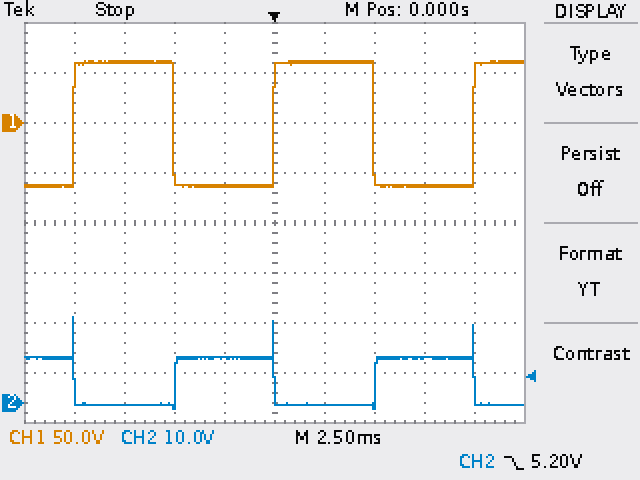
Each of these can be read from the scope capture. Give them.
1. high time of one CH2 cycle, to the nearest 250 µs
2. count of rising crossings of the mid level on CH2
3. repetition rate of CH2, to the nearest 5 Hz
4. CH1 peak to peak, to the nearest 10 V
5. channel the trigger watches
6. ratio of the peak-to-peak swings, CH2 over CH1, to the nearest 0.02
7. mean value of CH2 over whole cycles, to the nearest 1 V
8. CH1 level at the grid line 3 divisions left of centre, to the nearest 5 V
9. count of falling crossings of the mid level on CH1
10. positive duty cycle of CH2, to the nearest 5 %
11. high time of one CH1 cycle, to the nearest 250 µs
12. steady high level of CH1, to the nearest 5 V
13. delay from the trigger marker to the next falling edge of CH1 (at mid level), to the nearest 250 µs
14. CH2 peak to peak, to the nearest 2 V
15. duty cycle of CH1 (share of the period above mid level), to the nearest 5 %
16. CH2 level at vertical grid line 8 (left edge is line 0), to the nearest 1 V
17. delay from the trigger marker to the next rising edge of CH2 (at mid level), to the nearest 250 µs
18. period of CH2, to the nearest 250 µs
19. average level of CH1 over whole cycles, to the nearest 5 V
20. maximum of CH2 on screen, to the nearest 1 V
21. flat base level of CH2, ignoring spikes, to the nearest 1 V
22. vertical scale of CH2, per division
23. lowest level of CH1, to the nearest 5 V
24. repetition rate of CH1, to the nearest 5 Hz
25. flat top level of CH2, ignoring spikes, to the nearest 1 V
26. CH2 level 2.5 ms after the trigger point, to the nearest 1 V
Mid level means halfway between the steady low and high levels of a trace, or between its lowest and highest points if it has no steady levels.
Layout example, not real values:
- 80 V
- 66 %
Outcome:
- 5.00 ms
- 2
- 100 Hz
- 130 V
- CH2
- 0.14
- 4 V
- 60 V
- 2
- 50 %
- 5.00 ms
- 60 V
- 5.00 ms
- 18 V
- 50 %
- 9 V
- 5.00 ms
- 10.00 ms
- 0 V
- 17 V
- 0 V
- 10 V
- -65 V
- 100 Hz
- 9 V
- 0 V
